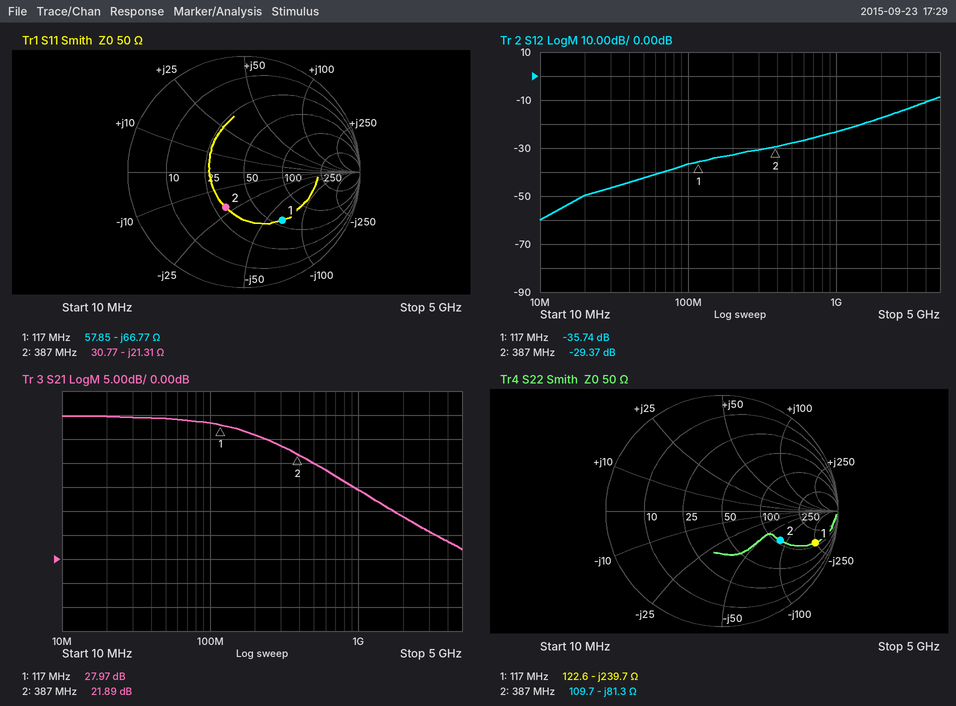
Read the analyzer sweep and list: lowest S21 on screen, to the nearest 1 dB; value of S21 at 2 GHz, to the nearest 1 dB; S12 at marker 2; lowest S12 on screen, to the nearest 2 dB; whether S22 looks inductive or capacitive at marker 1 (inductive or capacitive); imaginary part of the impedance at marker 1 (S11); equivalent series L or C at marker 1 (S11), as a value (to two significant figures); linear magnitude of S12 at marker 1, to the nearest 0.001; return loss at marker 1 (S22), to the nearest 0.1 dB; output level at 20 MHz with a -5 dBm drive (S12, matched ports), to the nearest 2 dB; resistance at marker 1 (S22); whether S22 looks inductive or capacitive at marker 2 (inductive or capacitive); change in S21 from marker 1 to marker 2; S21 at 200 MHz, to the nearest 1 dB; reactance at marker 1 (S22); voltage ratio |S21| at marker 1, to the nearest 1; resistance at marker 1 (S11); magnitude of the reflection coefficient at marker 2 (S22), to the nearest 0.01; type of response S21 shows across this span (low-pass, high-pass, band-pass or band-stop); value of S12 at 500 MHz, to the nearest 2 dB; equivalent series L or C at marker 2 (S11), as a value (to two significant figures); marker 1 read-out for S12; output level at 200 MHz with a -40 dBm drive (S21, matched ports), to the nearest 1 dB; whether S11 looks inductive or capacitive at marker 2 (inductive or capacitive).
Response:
2 dB
9 dB
-29.37 dB
-60 dB
capacitive
-66.77 Ω
20 pF
0.016
1.4 dB
-54 dBm
122.6 Ω
capacitive
-6.08 dB
26 dB
-239.7 Ω
25
57.85 Ω
0.56
low-pass
-28 dB
19 pF
-35.74 dB
-14 dBm
capacitive
